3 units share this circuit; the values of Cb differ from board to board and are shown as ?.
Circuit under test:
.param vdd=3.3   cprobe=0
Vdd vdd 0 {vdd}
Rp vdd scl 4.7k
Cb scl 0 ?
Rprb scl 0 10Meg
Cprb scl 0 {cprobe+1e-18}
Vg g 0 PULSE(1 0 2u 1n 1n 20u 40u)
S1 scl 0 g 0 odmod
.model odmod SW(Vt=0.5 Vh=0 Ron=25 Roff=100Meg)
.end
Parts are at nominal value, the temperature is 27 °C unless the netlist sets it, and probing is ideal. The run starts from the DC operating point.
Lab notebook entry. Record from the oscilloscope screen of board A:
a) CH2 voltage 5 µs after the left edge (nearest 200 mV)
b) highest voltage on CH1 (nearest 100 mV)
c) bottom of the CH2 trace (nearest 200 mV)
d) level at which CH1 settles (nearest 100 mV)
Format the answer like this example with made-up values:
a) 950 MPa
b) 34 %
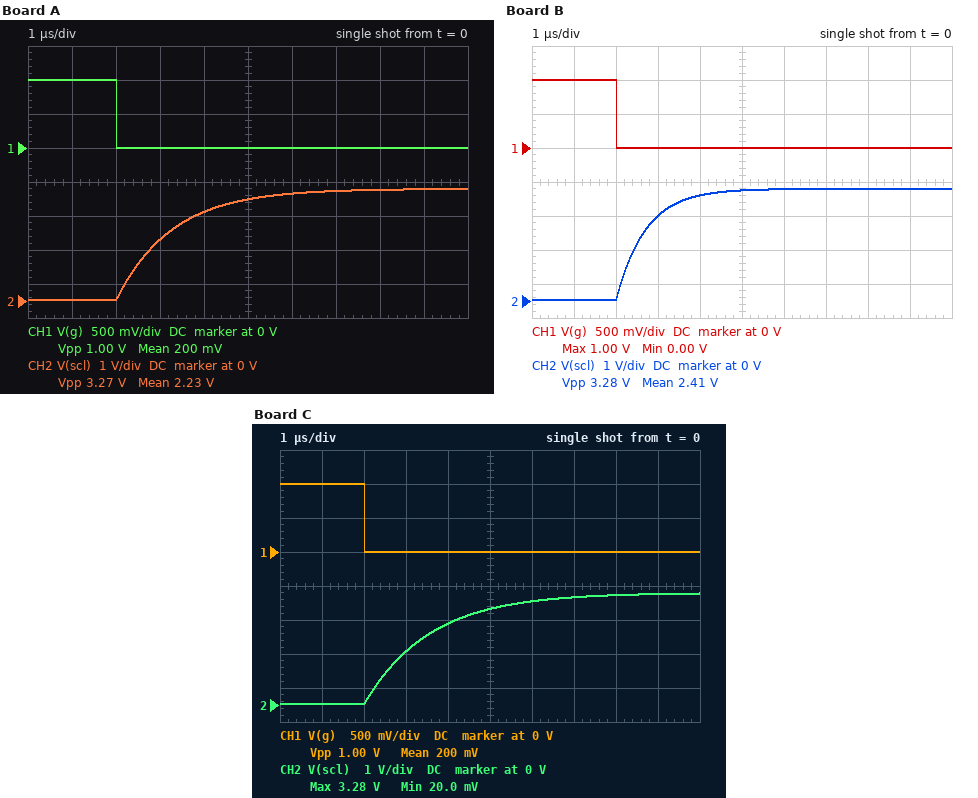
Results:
a) 3.0 V
b) 1.0 V
c) 0 V
d) 0 V
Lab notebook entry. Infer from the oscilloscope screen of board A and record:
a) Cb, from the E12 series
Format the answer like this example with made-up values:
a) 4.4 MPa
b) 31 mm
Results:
a) 270 pF
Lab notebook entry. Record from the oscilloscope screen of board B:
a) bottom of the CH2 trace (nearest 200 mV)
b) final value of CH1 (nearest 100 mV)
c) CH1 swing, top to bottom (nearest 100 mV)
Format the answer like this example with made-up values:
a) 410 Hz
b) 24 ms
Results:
a) 0 V
b) 0 V
c) 1.0 V
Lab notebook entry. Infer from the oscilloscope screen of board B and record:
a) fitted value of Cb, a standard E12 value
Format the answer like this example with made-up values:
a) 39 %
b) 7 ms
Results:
a) 150 pF
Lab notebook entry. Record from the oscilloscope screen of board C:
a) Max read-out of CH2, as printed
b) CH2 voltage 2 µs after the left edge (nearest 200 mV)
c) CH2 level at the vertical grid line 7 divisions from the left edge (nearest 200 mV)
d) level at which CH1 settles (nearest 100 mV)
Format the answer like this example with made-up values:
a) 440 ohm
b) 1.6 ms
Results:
a) 3.28 V
b) 0 V
c) 3.2 V
d) 0 V
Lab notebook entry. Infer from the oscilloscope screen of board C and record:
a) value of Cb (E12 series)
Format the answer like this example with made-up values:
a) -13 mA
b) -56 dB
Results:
a) 330 pF
